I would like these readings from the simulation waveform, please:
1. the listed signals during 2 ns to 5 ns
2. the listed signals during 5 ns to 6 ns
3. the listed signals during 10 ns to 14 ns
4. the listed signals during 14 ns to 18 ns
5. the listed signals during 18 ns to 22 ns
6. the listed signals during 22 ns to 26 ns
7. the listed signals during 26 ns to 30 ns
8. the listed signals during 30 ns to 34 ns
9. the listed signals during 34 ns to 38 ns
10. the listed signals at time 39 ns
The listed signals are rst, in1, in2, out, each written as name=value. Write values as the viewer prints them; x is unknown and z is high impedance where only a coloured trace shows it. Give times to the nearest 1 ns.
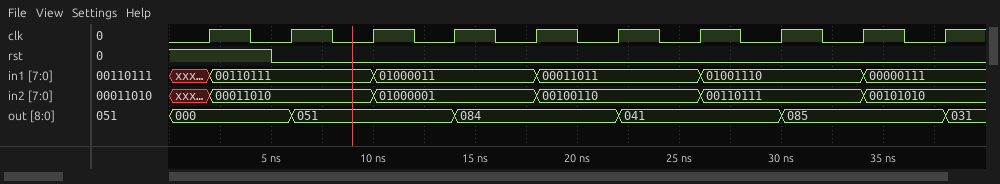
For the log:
rst=1, in1=00110111, in2=00011010, out=000
rst=0, in1=00110111, in2=00011010, out=000
rst=0, in1=01000011, in2=01000001, out=051
rst=0, in1=01000011, in2=01000001, out=084
rst=0, in1=00011011, in2=00100110, out=084
rst=0, in1=00011011, in2=00100110, out=041
rst=0, in1=01001110, in2=00110111, out=041
rst=0, in1=01001110, in2=00110111, out=085
rst=0, in1=00000111, in2=00101010, out=085
rst=0, in1=00000111, in2=00101010, out=031
